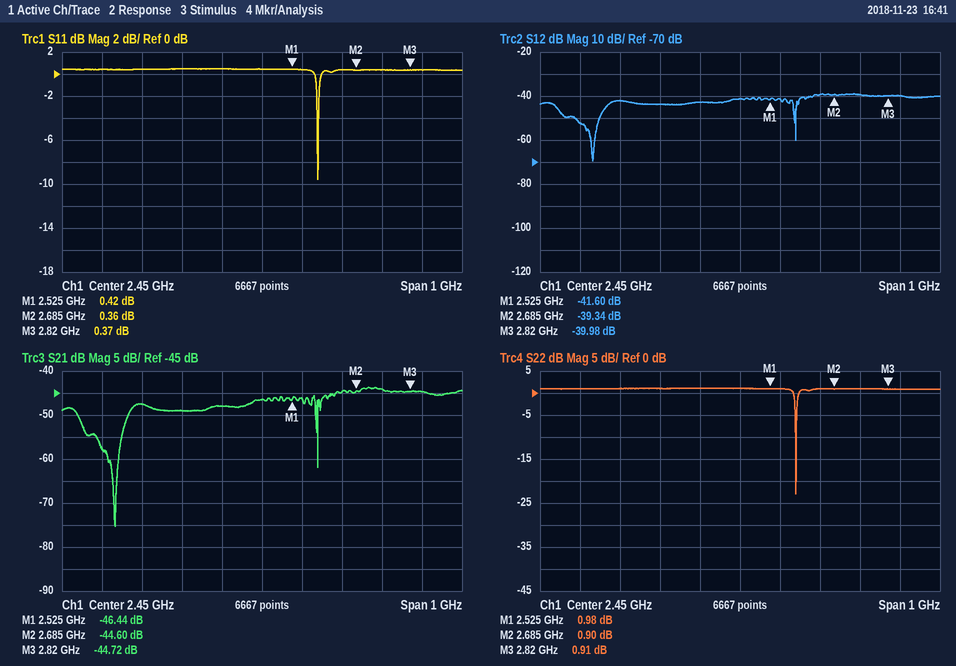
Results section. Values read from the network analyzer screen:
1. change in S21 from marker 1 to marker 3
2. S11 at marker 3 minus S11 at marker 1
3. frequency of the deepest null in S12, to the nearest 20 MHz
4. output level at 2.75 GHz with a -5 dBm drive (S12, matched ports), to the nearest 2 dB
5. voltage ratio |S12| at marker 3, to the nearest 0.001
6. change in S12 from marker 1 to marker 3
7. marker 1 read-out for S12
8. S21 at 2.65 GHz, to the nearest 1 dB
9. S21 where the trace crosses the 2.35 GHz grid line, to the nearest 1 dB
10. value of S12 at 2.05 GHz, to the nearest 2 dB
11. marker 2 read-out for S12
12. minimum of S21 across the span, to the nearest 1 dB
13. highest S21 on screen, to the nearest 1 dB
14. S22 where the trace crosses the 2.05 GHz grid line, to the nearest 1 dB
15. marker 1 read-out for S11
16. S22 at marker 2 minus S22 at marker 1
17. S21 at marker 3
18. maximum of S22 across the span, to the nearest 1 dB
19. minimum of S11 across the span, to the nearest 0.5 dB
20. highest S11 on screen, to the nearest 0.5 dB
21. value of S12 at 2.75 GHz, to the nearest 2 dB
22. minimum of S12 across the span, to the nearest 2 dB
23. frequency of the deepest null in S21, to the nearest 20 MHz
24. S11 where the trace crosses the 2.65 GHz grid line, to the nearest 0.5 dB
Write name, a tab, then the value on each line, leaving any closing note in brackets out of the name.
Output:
change in S21 from marker 1 to marker 3	1.72 dB
S11 at marker 3 minus S11 at marker 1	-0.05 dB
frequency of the deepest null in S12, to the nearest 20 MHz	2.08 GHz
output level at 2.75 GHz with a -5 dBm drive (S12, matched ports), to the nearest 2 dB	-44 dBm
voltage ratio |S12| at marker 3, to the nearest 0.001	0.010
change in S12 from marker 1 to marker 3	1.62 dB
marker 1 read-out for S12	-41.60 dB
S21 at 2.65 GHz, to the nearest 1 dB	-45 dB
S21 where the trace crosses the 2.35 GHz grid line, to the nearest 1 dB	-48 dB
value of S12 at 2.05 GHz, to the nearest 2 dB	-52 dB
marker 2 read-out for S12	-39.34 dB
minimum of S21 across the span, to the nearest 1 dB	-75 dB
highest S21 on screen, to the nearest 1 dB	-44 dB
S22 where the trace crosses the 2.05 GHz grid line, to the nearest 1 dB	1 dB
marker 1 read-out for S11	0.42 dB
S22 at marker 2 minus S22 at marker 1	-0.08 dB
S21 at marker 3	-44.72 dB
maximum of S22 across the span, to the nearest 1 dB	1 dB
minimum of S11 across the span, to the nearest 0.5 dB	-9.5 dB
highest S11 on screen, to the nearest 0.5 dB	0.5 dB
value of S12 at 2.75 GHz, to the nearest 2 dB	-40 dB
minimum of S12 across the span, to the nearest 2 dB	-70 dB
frequency of the deepest null in S21, to the nearest 20 MHz	2.08 GHz
S11 where the trace crosses the 2.65 GHz grid line, to the nearest 0.5 dB	0.5 dB
